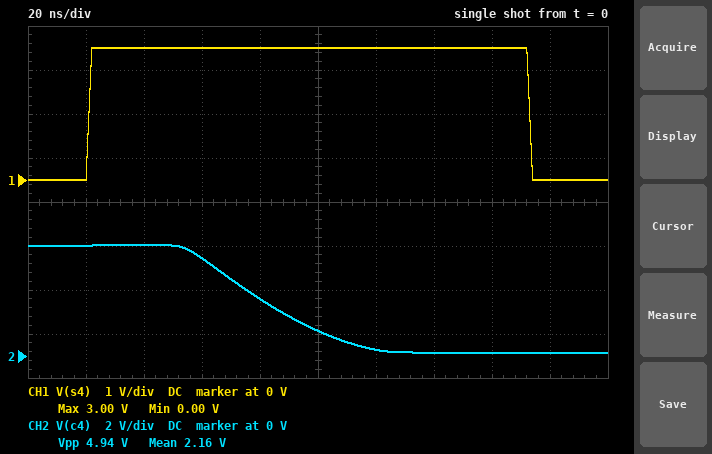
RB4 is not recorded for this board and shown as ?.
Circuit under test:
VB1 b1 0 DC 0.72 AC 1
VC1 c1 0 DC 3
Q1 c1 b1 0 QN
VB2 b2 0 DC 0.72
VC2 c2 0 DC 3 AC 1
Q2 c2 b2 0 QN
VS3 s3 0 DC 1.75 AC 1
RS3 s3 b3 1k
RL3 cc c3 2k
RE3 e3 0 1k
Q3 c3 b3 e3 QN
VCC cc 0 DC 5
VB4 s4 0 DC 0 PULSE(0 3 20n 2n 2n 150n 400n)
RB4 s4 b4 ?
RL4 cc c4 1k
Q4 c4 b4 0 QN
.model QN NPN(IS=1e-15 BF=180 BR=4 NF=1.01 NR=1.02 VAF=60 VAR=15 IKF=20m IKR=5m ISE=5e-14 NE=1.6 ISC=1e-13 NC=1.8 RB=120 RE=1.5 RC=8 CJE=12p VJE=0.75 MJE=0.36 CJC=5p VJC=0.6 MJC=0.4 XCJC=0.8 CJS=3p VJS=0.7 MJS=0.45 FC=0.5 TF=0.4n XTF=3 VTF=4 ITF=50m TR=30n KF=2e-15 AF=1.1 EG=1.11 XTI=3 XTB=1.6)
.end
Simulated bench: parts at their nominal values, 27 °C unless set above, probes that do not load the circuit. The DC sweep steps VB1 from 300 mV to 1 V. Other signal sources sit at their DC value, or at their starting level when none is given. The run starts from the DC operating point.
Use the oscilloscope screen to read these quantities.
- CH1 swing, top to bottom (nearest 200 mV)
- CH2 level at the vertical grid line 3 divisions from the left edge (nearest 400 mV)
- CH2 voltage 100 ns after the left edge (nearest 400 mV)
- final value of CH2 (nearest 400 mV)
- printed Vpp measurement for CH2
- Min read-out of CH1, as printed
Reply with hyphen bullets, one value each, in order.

- 3.0 V
- 4.4 V
- 1.2 V
- 0 V
- 4.94 V
- 0.00 V
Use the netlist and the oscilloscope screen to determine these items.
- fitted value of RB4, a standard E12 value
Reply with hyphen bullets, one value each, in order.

- 6.8 kΩ
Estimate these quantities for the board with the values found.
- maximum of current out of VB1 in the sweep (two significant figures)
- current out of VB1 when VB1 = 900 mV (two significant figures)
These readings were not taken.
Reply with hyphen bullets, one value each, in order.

- 750 µA
- 320 µA
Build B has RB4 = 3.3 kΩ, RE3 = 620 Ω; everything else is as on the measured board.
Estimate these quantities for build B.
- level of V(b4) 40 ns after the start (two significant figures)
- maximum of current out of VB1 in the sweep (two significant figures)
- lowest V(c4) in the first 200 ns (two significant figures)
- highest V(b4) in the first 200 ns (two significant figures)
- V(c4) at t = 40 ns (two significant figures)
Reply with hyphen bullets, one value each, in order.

- 800 mV
- 750 µA
- 89 mV
- 870 mV
- 4.6 V
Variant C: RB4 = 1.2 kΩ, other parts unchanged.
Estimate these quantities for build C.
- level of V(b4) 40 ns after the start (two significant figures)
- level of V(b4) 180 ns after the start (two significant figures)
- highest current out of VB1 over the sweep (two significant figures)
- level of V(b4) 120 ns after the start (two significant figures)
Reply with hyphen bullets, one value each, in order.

- 960 mV
- 720 mV
- 750 µA
- 1.0 V
